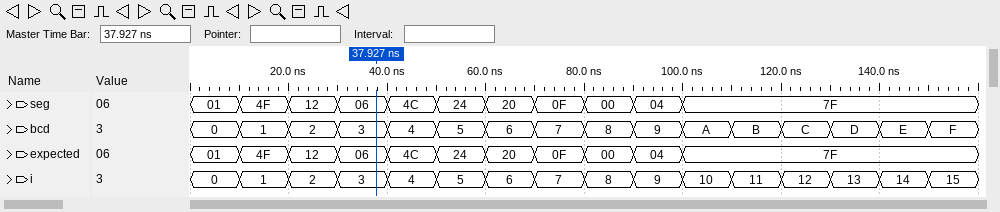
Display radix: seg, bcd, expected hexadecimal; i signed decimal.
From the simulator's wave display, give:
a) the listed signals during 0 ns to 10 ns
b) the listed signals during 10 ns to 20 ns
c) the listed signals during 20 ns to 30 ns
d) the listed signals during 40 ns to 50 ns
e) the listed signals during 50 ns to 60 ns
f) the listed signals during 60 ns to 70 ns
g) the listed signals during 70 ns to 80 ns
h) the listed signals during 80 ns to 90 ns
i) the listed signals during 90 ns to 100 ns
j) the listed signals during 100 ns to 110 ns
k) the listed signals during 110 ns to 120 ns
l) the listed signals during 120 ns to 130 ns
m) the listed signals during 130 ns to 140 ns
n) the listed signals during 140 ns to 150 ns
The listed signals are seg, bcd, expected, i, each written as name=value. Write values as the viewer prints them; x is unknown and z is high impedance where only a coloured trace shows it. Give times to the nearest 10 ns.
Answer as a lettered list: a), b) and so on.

a) seg=01, bcd=0, expected=01, i=0
b) seg=4F, bcd=1, expected=4F, i=1
c) seg=12, bcd=2, expected=12, i=2
d) seg=4C, bcd=4, expected=4C, i=4
e) seg=24, bcd=5, expected=24, i=5
f) seg=20, bcd=6, expected=20, i=6
g) seg=0F, bcd=7, expected=0F, i=7
h) seg=00, bcd=8, expected=00, i=8
i) seg=04, bcd=9, expected=04, i=9
j) seg=7F, bcd=A, expected=7F, i=10
k) seg=7F, bcd=B, expected=7F, i=11
l) seg=7F, bcd=C, expected=7F, i=12
m) seg=7F, bcd=D, expected=7F, i=13
n) seg=7F, bcd=E, expected=7F, i=14
